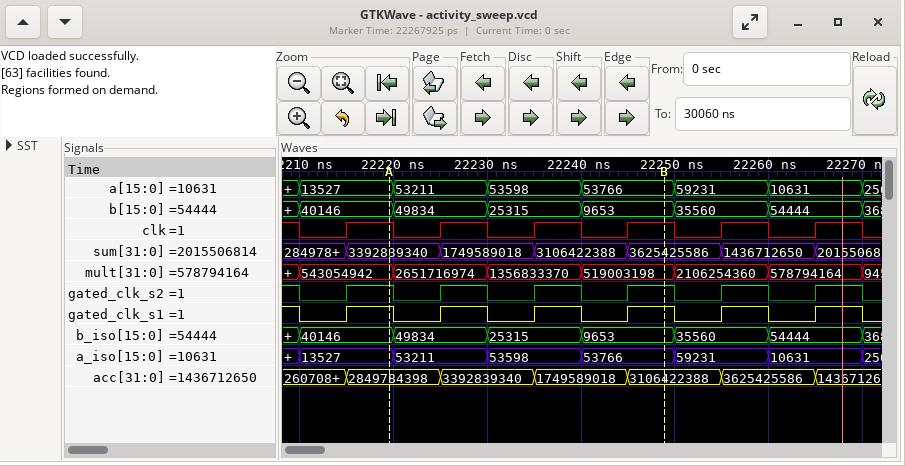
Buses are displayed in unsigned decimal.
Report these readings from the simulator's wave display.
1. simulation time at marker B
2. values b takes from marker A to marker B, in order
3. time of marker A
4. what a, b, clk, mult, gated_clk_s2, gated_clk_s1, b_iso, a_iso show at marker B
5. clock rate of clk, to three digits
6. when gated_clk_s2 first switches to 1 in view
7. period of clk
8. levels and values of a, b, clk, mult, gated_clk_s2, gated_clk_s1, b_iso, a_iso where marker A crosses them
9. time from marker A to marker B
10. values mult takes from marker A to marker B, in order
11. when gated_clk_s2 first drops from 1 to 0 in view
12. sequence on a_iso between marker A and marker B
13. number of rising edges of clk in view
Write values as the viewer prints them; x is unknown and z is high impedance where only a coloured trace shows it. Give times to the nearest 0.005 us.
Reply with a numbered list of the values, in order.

1. 22.25 us
2. 40146, 49834, 25315, 9653
3. 22.22 us
4. a=53766, b=9653, clk=1, mult=519003198, gated_clk_s2=1, gated_clk_s1=1, b_iso=9653, a_iso=53766
5. 100 MHz
6. 22.215 us
7. 0.01 us
8. a=13527, b=40146, clk=1, mult=543054942, gated_clk_s2=1, gated_clk_s1=1, b_iso=40146, a_iso=13527
9. 0.03 us
10. 543054942, 2651716974, 1356833370, 519003198
11. 22.21 us
12. 13527, 53211, 53598, 53766
13. 6
